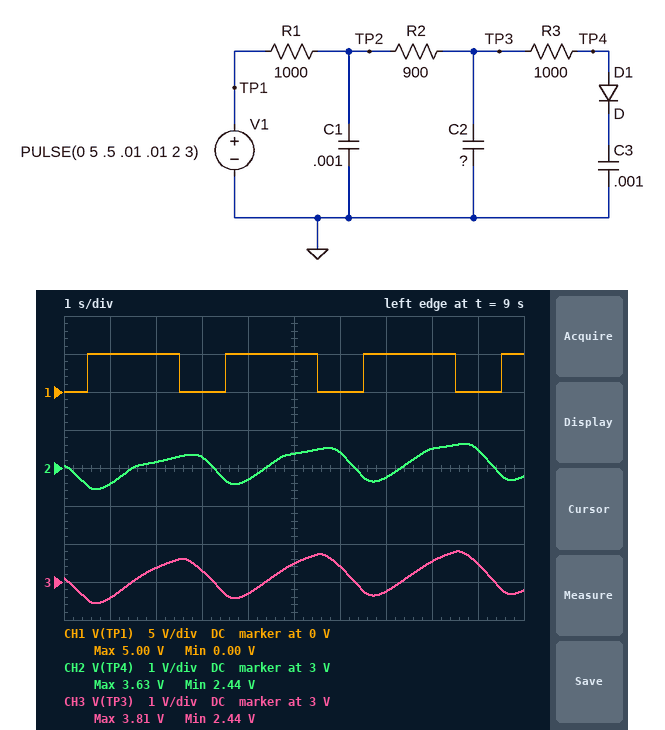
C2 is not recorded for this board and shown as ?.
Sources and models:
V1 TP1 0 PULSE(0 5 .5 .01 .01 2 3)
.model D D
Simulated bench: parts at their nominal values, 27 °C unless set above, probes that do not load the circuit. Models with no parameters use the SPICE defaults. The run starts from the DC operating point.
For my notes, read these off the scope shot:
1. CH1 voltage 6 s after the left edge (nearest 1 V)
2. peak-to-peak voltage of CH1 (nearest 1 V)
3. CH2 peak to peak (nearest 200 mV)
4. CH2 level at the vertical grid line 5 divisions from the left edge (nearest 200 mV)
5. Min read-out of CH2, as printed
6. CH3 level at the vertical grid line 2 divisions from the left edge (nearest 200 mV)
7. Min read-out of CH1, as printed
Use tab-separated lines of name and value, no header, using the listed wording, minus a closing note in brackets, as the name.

CH1 voltage 6 s after the left edge	0 V
peak-to-peak voltage of CH1	5 V
CH2 peak to peak	1.2 V
CH2 level at the vertical grid line 5 divisions from the left edge	3.4 V
Min read-out of CH2, as printed	2.44 V
CH3 level at the vertical grid line 2 divisions from the left edge	3.4 V
Min read-out of CH1, as printed	0.00 V
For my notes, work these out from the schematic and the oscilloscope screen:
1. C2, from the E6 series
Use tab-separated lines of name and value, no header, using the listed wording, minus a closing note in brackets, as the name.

C2, from the E6 series	680 µF
